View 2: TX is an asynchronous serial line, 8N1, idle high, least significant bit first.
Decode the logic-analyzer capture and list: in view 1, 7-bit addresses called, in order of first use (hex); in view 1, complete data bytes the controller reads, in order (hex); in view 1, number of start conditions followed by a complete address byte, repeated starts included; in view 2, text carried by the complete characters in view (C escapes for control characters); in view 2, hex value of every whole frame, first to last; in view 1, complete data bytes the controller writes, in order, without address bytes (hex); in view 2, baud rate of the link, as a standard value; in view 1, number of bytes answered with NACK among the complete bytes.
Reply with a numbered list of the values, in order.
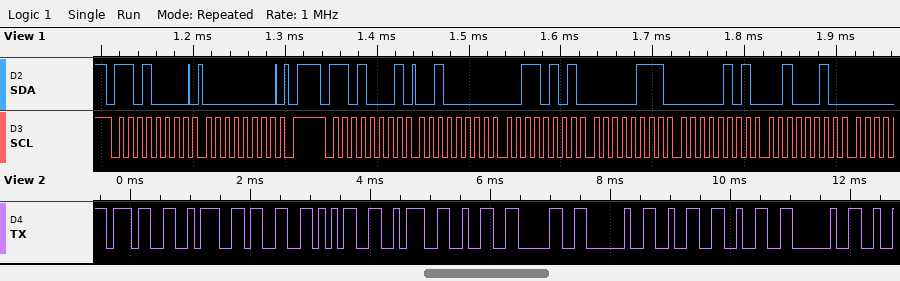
1. 0x68
2. 20 35 07 05 22
3. 2
4. "7:35:20 22 "
5. 37 3A 33 35 3A 32 30 20 32 32 20
6. 00
7. 9600 baud
8. 0
